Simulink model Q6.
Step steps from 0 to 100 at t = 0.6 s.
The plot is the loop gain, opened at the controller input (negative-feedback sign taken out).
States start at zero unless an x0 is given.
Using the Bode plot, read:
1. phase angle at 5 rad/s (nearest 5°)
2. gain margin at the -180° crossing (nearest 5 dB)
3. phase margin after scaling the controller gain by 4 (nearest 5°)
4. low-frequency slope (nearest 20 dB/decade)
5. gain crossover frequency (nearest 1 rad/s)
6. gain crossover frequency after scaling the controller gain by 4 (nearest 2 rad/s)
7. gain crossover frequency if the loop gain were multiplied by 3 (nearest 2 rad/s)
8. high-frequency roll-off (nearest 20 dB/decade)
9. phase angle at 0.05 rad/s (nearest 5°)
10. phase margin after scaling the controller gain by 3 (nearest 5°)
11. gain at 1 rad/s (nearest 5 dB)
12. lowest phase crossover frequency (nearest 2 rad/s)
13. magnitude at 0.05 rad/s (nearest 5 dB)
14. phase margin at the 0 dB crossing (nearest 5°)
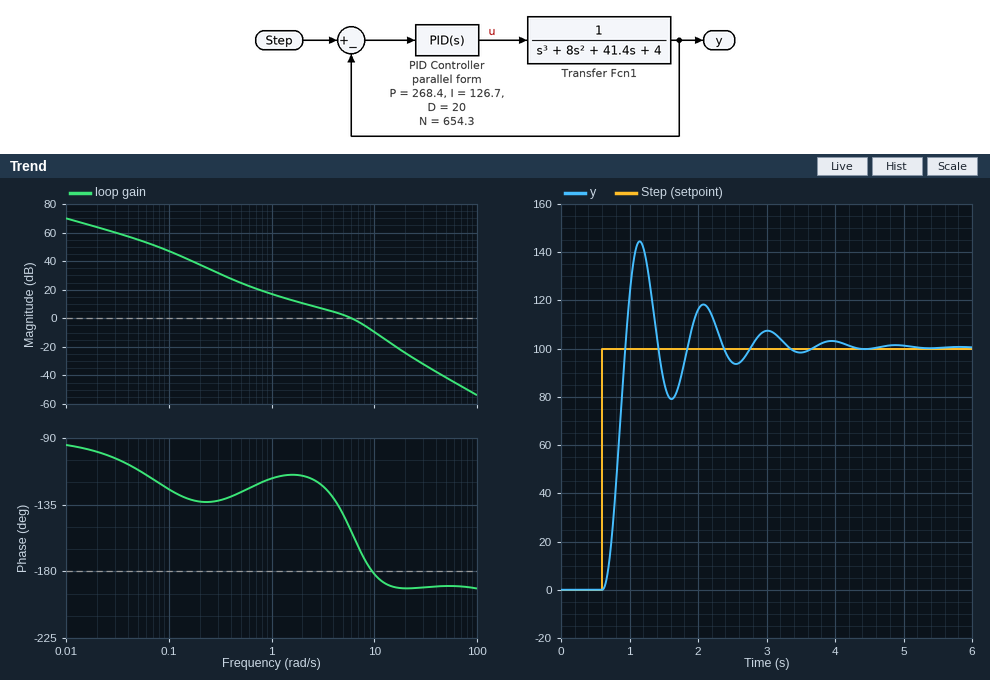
-140°
10 dB
-5°
-20 dB/decade
6 rad/s
12 rad/s
10 rad/s
-40 dB/decade
-110°
0°
15 dB
10 rad/s
55 dB
25°
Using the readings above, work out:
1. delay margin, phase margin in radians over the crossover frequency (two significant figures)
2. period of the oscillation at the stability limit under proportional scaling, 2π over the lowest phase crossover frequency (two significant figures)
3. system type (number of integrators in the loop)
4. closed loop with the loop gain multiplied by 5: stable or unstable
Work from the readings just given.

0.073 s
0.63 s
1
unstable
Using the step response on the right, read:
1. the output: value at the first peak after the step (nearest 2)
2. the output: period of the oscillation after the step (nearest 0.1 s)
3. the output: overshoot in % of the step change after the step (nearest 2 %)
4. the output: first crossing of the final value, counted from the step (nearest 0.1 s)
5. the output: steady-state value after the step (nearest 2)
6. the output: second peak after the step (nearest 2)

144
0.9 s
44 %
0.3 s
100
118
